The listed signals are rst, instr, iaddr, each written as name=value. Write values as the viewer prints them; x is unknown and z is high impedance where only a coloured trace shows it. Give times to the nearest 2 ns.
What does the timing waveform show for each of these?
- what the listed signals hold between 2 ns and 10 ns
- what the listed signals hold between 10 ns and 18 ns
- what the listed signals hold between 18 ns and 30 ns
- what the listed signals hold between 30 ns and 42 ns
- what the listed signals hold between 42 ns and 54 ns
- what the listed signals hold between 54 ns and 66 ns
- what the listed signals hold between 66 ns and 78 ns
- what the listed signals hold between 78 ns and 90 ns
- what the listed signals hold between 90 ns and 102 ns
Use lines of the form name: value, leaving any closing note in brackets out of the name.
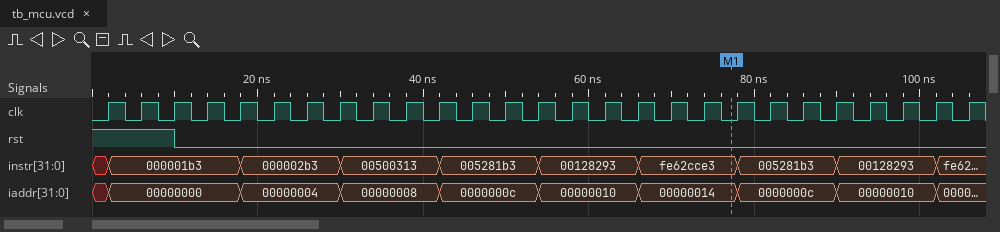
what the listed signals hold between 2 ns and 10 ns: rst=1, instr=000001b3, iaddr=00000000
what the listed signals hold between 10 ns and 18 ns: rst=0, instr=000001b3, iaddr=00000000
what the listed signals hold between 18 ns and 30 ns: rst=0, instr=000002b3, iaddr=00000004
what the listed signals hold between 30 ns and 42 ns: rst=0, instr=00500313, iaddr=00000008
what the listed signals hold between 42 ns and 54 ns: rst=0, instr=005281b3, iaddr=0000000c
what the listed signals hold between 54 ns and 66 ns: rst=0, instr=00128293, iaddr=00000010
what the listed signals hold between 66 ns and 78 ns: rst=0, instr=fe62cce3, iaddr=00000014
what the listed signals hold between 78 ns and 90 ns: rst=0, instr=005281b3, iaddr=0000000c
what the listed signals hold between 90 ns and 102 ns: rst=0, instr=00128293, iaddr=00000010
